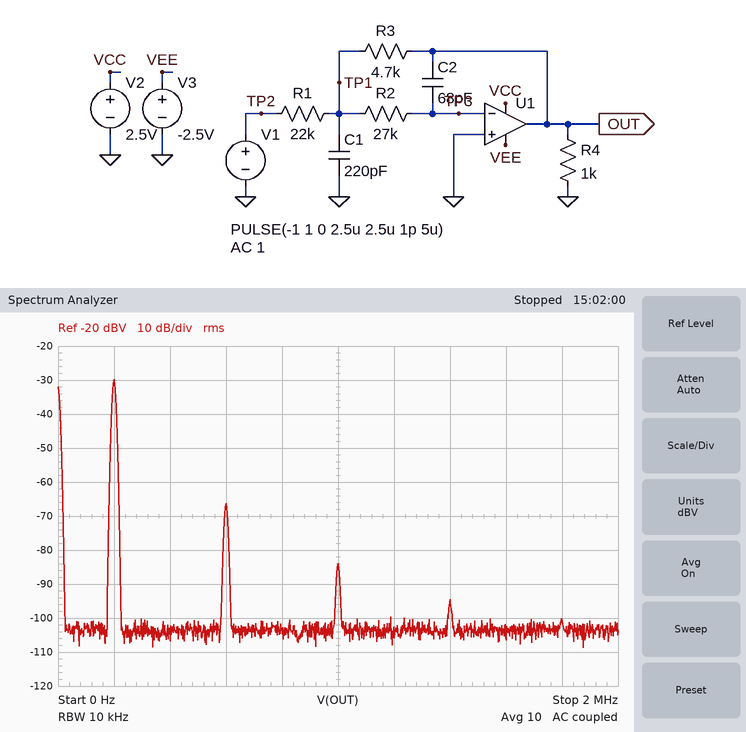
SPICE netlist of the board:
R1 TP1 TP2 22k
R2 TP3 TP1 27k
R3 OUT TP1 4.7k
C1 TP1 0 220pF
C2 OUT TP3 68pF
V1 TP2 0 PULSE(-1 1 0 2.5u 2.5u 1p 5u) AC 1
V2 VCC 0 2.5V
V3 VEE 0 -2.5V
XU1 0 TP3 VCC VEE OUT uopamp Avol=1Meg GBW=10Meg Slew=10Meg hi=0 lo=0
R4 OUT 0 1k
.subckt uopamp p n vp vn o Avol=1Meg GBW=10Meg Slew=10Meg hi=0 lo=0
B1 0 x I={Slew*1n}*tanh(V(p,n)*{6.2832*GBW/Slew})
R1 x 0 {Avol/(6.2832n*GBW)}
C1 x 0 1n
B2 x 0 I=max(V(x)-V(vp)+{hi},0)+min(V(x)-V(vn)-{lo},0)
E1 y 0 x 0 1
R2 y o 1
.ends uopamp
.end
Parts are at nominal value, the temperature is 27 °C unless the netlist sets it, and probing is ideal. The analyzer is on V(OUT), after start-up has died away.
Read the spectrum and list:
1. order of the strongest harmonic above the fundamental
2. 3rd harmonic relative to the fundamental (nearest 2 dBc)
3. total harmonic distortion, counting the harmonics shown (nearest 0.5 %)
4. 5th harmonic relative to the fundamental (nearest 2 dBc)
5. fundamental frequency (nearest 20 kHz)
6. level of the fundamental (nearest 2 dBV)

3
-36 dBc
1.5 %
-54 dBc
200 kHz
-30 dBV
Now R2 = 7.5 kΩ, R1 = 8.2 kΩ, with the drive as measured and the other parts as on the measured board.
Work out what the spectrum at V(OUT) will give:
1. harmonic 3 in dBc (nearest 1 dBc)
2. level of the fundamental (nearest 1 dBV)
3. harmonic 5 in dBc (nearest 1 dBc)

-34 dBc
-13 dBV
-52 dBc
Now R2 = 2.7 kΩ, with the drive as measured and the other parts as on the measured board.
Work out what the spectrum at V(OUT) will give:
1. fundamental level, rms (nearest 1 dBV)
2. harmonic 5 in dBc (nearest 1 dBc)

-18 dBV
-46 dBc
